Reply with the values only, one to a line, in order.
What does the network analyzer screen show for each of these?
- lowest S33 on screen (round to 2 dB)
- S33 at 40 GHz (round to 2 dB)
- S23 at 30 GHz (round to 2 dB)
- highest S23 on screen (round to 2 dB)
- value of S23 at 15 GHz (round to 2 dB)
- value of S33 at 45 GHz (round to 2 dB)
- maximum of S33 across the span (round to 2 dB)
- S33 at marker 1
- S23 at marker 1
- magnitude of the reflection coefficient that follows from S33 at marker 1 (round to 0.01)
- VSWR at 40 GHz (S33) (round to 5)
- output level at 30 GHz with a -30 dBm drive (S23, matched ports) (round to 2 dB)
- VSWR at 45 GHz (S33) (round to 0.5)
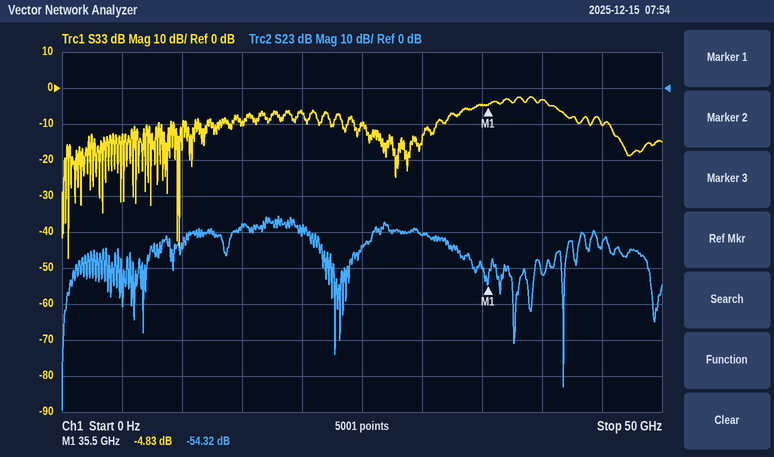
-48 dB
-4 dB
-40 dB
-36 dB
-38 dB
-10 dB
-2 dB
-4.83 dB
-54.32 dB
0.57
5
-70 dBm
2.0
